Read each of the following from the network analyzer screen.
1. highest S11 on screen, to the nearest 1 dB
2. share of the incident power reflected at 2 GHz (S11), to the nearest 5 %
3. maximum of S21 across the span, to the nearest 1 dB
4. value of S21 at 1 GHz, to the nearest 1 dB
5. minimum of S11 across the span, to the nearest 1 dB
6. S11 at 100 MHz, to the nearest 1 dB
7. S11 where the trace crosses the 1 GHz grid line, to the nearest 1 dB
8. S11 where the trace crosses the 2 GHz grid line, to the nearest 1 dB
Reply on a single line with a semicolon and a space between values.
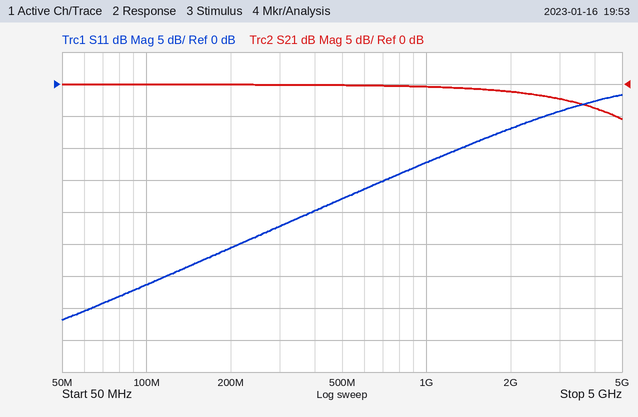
-2 dB; 20 %; 0 dB; 0 dB; -37 dB; -31 dB; -12 dB; -7 dB
